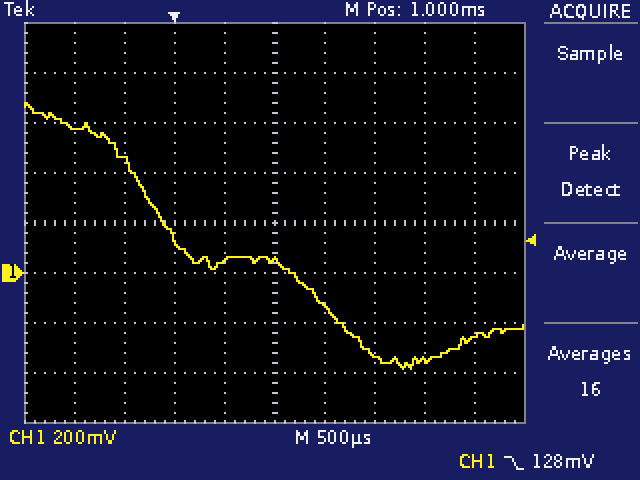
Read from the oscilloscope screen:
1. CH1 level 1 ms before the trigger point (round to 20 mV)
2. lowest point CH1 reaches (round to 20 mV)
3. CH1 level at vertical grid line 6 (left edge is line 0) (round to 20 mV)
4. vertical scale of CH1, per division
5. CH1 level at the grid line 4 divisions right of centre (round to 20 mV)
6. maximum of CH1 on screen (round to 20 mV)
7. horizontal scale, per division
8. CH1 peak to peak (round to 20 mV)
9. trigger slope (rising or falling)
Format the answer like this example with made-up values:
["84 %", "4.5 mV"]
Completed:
["580 mV", "-380 mV", "-140 mV", "200 mV", "-260 mV", "680 mV", "500 µs", "1.06 V", "falling"]
